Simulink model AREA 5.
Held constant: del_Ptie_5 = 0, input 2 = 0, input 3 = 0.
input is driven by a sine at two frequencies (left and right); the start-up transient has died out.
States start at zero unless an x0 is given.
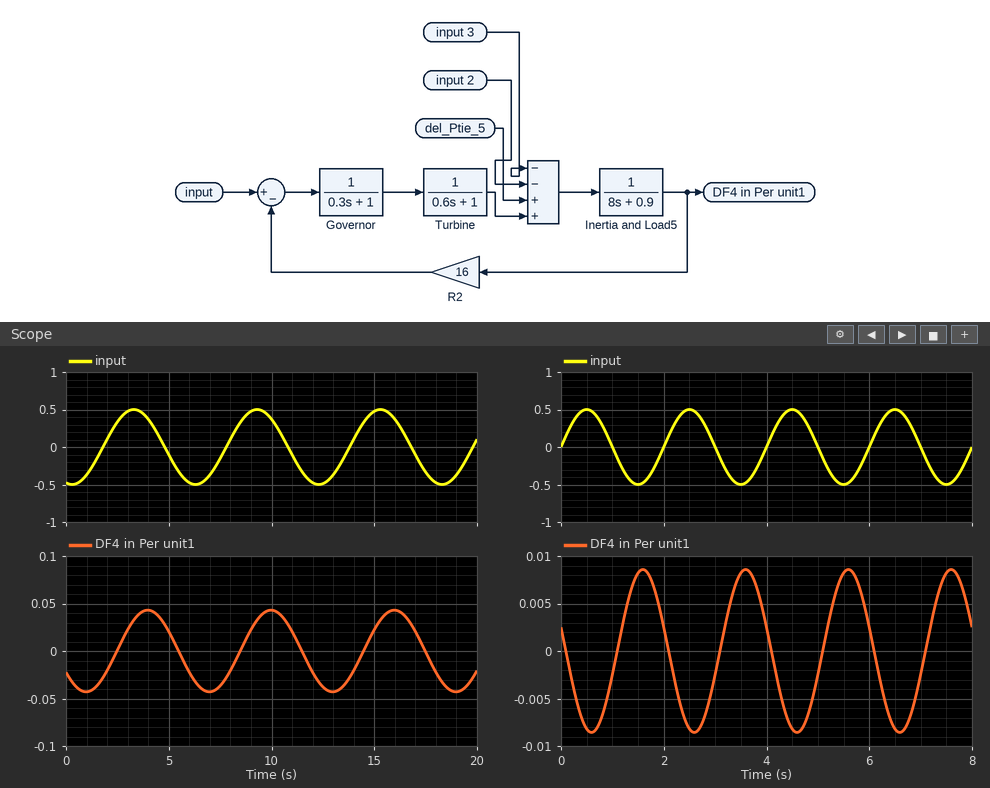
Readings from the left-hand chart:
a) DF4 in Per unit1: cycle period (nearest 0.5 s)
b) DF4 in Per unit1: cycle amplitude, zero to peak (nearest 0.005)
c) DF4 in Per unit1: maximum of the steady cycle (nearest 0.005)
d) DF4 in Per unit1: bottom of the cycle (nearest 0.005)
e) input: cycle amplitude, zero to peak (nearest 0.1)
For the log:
6.0 s
0.045
0.045
-0.045
0.5
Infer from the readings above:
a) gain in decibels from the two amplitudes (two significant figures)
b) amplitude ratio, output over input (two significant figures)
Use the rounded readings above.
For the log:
-21 dB
0.090
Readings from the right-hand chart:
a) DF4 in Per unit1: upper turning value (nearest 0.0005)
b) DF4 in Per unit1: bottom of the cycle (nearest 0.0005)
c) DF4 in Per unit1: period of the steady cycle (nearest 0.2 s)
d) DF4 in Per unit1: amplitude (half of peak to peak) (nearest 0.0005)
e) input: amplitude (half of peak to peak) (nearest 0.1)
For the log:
0.0085
-0.0085
2.0 s
0.0085
0.5
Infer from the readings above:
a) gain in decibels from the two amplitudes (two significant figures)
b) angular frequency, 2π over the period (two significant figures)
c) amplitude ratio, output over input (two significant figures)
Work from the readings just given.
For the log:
-35 dB
3.1 rad/s
0.017
